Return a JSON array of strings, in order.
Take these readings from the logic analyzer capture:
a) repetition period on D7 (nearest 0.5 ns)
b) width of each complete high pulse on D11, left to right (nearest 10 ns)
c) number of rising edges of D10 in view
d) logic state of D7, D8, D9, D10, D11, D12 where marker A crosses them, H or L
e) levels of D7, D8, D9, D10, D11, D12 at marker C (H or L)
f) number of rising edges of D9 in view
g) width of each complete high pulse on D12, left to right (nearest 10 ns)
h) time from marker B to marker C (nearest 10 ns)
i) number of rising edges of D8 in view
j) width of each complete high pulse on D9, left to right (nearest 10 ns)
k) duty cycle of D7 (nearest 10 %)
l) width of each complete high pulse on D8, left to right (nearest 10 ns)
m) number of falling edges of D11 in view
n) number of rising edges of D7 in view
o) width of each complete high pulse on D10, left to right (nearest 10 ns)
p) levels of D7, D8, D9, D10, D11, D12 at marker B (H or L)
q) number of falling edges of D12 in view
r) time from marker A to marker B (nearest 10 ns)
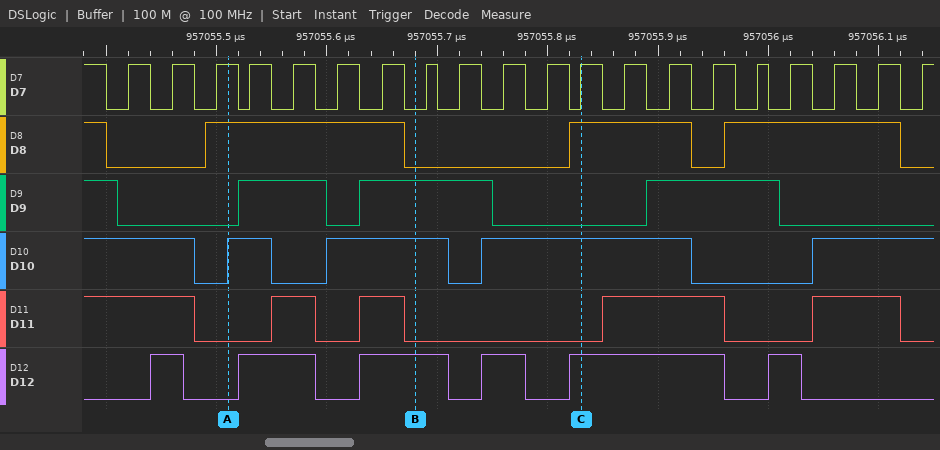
["38 ns", "40 ns, 40 ns, 110 ns, 80 ns", "4", "D7=H, D8=H, D9=L, D10=H, D11=L, D12=L", "D7=H, D8=H, D9=L, D10=H, D11=L, D12=H", "3", "30 ns, 70 ns, 80 ns, 40 ns, 140 ns, 30 ns", "150 ns", "3", "80 ns, 120 ns, 120 ns", "50 %", "180 ns, 110 ns, 160 ns", "5", "20", "40 ns, 110 ns, 190 ns", "D7=L, D8=L, D9=H, D10=H, D11=L, D12=H", "6", "170 ns"]
